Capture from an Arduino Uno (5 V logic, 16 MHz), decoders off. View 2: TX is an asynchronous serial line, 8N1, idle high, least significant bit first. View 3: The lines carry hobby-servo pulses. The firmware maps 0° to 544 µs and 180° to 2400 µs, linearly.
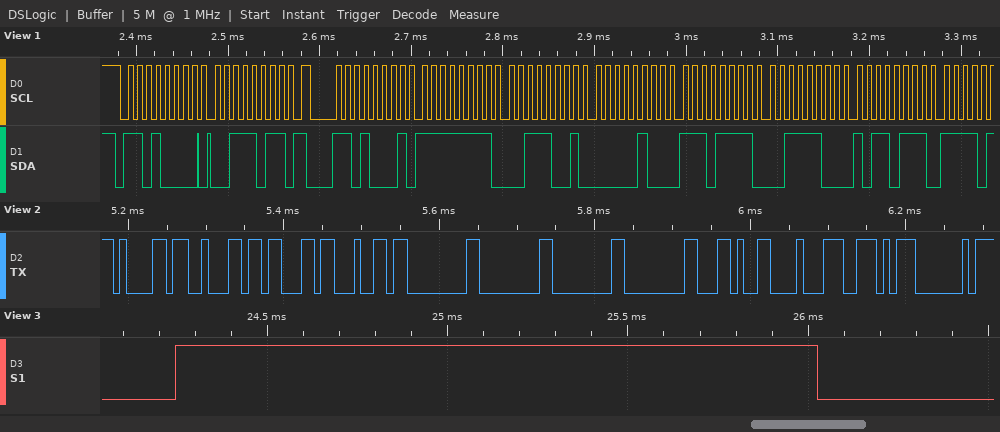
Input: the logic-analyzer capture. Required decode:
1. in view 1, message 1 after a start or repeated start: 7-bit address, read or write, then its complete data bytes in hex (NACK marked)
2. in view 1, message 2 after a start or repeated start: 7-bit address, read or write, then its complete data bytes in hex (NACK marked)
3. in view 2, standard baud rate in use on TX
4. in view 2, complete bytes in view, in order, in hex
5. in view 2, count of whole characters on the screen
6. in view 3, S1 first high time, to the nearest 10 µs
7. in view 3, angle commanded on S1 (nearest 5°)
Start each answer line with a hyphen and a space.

- 0x68 write: 3B
- 0x68 read: FF 39 04 EF 3C B7
- 115200 baud
- 61 62 63 64 00 00 00 00 2C 88 AE 40
- 12
- 1780 µs
- 120°
